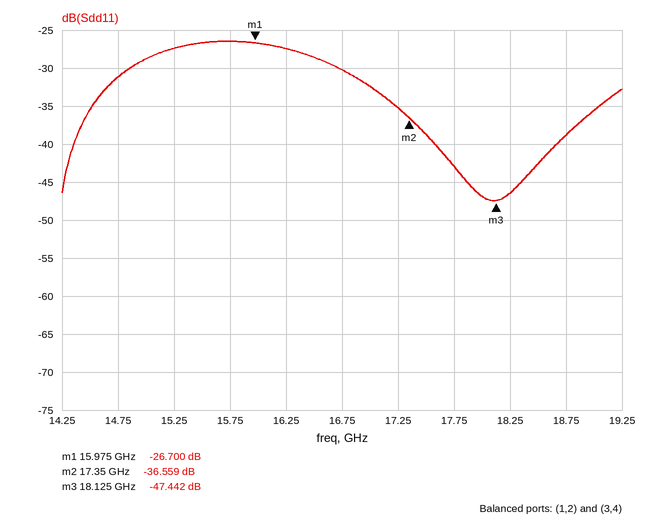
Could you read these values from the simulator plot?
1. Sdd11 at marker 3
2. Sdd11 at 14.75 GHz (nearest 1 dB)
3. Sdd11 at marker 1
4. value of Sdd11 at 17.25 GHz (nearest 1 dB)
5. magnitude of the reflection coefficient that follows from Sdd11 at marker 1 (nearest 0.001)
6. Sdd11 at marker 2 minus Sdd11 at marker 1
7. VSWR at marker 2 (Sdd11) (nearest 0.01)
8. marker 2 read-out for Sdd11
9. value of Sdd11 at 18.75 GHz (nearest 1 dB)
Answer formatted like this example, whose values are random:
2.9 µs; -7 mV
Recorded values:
-47.442 dB; -31 dB; -26.700 dB; -35 dB; 0.046; -9.859 dB; 1.03; -36.559 dB; -39 dB
